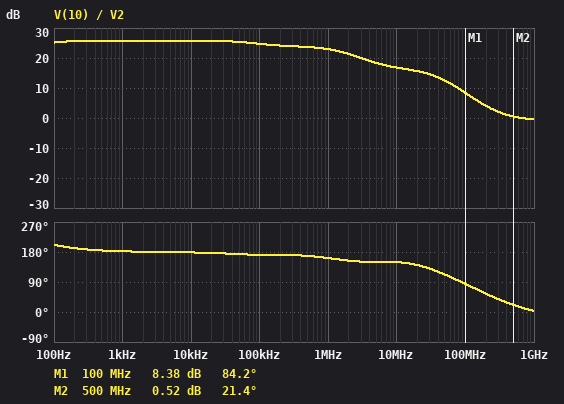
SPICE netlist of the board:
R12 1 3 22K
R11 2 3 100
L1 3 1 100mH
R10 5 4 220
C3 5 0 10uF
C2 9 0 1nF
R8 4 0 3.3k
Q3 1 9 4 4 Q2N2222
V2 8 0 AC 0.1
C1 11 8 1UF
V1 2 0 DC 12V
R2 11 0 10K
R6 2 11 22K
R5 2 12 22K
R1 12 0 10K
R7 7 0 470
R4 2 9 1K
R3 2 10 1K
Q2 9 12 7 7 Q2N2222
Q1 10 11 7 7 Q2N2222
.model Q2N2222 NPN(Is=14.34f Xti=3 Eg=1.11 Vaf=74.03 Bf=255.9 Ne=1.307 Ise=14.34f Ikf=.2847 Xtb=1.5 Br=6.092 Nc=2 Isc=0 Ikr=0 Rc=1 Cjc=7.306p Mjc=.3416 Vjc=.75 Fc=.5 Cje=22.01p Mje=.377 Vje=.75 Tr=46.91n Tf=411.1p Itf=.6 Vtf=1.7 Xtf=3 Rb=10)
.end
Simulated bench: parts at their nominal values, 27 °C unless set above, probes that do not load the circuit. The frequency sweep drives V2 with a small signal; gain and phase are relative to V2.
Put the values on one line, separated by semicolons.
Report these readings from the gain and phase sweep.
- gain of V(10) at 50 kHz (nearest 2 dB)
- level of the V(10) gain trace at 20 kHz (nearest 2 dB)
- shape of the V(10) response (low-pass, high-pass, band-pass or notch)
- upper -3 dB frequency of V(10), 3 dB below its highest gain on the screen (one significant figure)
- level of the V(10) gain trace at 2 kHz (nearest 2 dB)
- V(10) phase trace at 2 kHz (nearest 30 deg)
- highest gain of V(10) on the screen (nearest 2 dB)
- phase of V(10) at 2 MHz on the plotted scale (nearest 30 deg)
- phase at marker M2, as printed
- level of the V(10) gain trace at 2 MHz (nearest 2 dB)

26 dB; 26 dB; low-pass; 1 MHz; 26 dB; 180 deg; 26 dB; 150 deg; 21.4 deg; 22 dB
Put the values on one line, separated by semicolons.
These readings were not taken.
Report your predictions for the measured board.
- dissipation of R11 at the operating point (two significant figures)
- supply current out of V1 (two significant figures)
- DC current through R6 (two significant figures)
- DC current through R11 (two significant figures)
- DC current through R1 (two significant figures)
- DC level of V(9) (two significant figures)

610 µW; 9.5 mA; 380 µA; 2.5 mA; 360 µA; 8.9 V
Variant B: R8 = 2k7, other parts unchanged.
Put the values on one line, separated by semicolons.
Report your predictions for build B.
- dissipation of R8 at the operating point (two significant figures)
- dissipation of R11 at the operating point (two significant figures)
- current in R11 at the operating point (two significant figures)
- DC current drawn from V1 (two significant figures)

25 mW; 910 µW; 3.0 mA; 10 mA
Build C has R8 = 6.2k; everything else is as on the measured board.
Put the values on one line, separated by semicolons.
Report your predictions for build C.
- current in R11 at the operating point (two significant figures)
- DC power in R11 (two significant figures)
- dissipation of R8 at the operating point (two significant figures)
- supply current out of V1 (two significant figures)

1.3 mA; 170 µW; 11 mW; 8.3 mA
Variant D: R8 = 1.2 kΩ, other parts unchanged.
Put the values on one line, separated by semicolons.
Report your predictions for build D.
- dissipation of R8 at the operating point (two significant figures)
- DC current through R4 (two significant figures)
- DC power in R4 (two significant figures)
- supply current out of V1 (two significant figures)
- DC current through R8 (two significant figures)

55 mW; 3.2 mA; 10 mW; 14 mA; 6.8 mA
